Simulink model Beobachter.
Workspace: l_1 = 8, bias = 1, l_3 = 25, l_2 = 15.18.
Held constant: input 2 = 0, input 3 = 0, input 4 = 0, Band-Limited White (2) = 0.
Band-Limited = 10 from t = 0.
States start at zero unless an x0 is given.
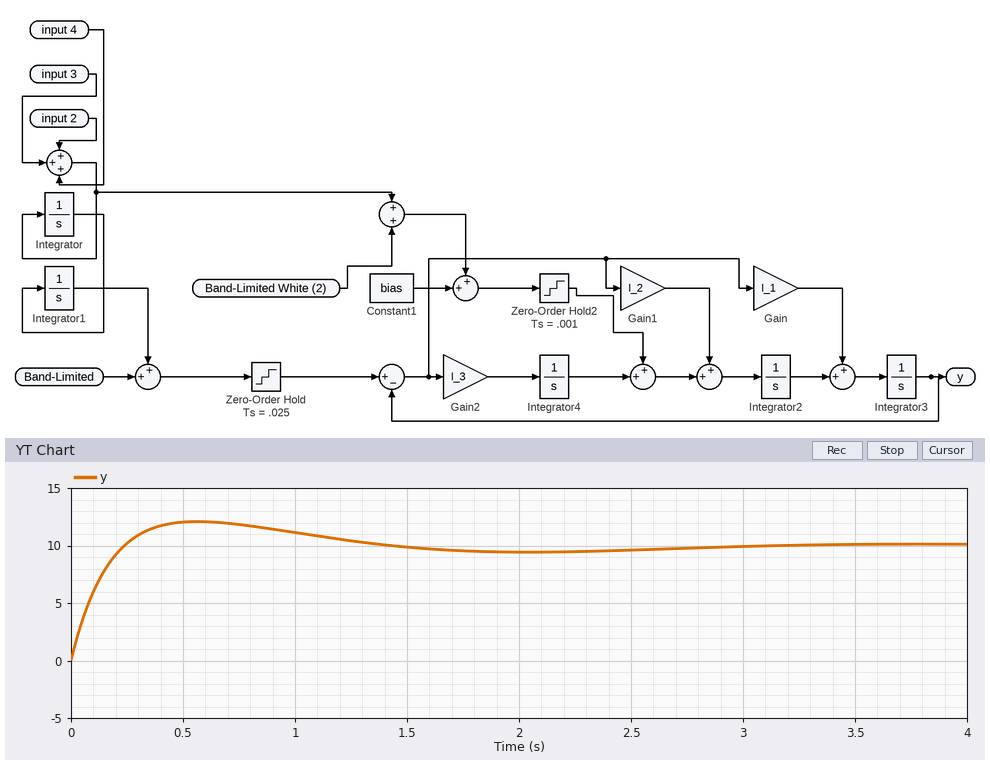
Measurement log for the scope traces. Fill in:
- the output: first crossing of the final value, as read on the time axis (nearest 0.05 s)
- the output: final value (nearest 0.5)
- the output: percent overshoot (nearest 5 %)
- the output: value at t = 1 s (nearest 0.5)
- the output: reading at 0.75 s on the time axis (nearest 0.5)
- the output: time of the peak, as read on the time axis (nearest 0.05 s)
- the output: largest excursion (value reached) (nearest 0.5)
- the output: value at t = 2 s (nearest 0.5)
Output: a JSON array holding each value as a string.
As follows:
["0.25 s", "10.0", "20 %", "11.0", "12.0", "0.55 s", "12.0", "9.5"]
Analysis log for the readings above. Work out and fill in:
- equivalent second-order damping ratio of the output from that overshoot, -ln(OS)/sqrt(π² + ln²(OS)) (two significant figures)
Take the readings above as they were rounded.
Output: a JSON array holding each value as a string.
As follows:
["0.46"]
